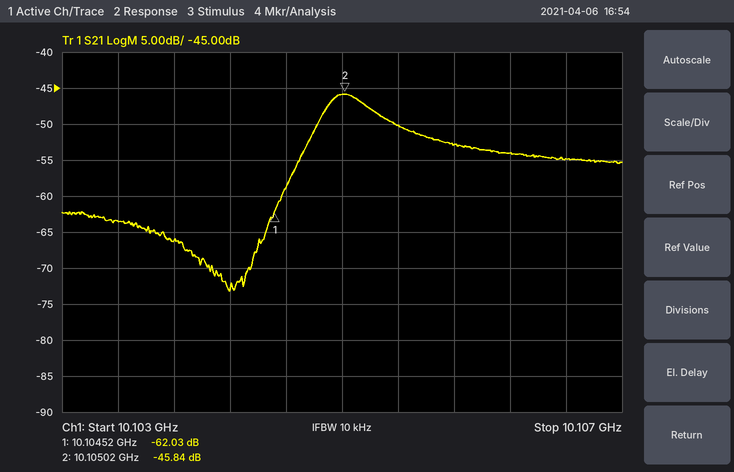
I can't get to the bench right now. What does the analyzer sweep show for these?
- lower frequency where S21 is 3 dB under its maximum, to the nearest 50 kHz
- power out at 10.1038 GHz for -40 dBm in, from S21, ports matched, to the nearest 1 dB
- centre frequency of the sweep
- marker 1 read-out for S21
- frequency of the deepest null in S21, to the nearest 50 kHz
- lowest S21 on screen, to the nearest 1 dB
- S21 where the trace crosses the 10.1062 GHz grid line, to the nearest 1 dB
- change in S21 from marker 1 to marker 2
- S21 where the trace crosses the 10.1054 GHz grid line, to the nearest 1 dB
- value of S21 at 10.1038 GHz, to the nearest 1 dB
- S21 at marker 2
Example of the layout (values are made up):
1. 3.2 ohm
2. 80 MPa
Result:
1. 10.10485 GHz
2. -106 dBm
3. 10.105 GHz
4. -62.03 dB
5. 10.10420 GHz
6. -73 dB
7. -54 dB
8. 16.19 dB
9. -50 dB
10. -66 dB
11. -45.84 dB
